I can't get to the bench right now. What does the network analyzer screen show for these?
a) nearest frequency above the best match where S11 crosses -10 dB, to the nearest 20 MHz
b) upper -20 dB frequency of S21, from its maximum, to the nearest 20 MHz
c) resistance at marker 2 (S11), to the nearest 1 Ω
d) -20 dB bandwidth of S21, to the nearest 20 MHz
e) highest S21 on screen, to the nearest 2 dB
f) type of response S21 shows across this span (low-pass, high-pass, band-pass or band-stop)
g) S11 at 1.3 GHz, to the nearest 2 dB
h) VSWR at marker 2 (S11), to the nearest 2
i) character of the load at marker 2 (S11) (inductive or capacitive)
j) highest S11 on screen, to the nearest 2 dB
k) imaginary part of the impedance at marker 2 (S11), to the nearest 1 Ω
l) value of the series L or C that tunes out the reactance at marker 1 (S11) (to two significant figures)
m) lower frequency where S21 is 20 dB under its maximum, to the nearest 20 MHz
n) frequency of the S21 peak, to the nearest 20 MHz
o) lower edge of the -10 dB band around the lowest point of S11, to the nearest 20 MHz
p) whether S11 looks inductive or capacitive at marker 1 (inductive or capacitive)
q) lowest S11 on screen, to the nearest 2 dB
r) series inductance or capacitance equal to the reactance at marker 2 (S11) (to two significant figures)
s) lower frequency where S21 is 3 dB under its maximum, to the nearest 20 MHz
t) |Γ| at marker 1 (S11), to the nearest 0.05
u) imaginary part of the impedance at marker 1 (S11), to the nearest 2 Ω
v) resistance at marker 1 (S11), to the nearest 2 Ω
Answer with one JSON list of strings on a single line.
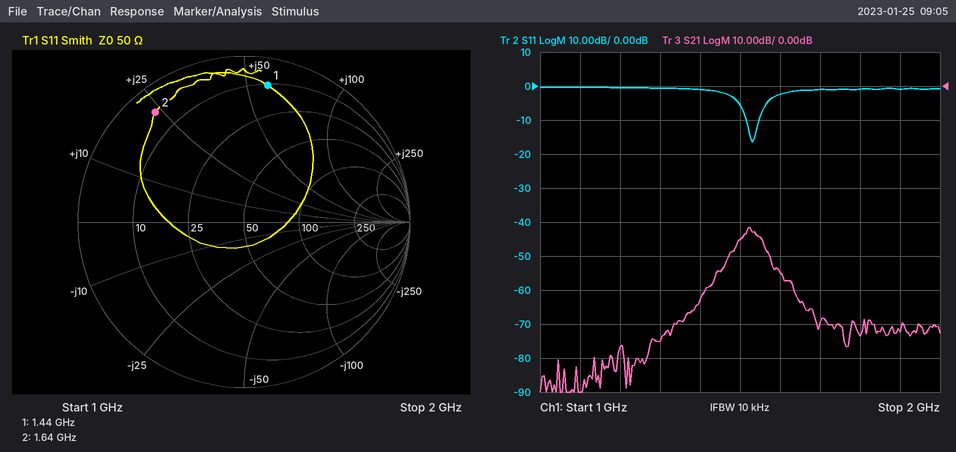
["1.54 GHz", "1.64 GHz", "5 Ω", "240 MHz", "-42 dB", "band-pass", "0 dB", "12", "inductive", "0 dB", "+24 Ω", "1.9 pF", "1.40 GHz", "1.52 GHz", "1.52 GHz", "inductive", "-16 dB", "2.3 nH", "1.50 GHz", "0.85", "+58 Ω", "10 Ω"]
